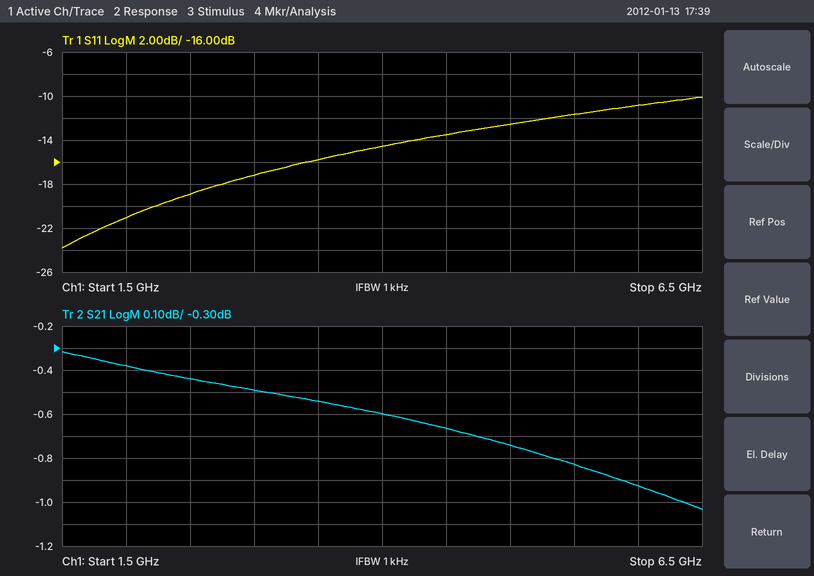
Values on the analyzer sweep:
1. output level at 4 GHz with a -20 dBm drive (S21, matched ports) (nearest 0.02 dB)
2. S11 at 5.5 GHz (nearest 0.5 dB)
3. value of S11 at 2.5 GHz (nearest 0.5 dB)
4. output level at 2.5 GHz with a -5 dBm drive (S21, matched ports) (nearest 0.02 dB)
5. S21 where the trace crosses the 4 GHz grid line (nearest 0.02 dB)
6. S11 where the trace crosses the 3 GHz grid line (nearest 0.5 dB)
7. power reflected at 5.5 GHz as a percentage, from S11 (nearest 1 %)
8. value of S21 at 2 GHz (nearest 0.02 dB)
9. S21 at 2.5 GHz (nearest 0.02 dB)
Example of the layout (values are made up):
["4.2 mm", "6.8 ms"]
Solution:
["-20.60 dBm", "-11.5 dB", "-19.0 dB", "-5.44 dBm", "-0.60 dB", "-17.0 dB", "7 %", "-0.38 dB", "-0.44 dB"]
